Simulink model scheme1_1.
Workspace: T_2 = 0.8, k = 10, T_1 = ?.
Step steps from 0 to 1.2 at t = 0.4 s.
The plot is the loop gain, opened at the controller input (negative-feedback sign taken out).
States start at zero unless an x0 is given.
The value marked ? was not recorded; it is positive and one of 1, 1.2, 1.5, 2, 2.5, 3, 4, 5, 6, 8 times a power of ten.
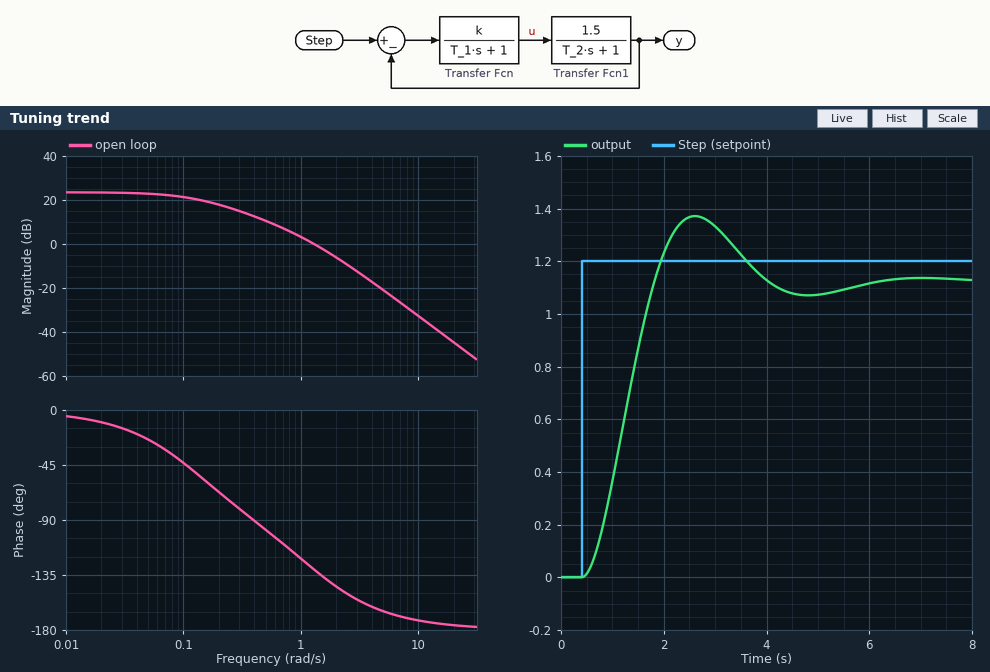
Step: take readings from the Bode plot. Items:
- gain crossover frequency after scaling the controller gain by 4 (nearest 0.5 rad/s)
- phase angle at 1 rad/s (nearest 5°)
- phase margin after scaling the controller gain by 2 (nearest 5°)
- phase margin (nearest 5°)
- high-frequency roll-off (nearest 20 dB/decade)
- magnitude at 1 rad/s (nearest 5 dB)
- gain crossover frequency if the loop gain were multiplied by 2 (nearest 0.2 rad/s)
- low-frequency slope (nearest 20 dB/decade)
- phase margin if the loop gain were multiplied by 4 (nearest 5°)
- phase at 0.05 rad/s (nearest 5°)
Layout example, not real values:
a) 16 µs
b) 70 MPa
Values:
a) 3.0 rad/s
b) -120°
c) 35°
d) 50°
e) -40 dB/decade
f) 5 dB
g) 2.0 rad/s
h) 0 dB/decade
i) 25°
j) -25°
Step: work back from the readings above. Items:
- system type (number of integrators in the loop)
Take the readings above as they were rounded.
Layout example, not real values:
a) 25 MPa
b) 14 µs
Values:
a) 0
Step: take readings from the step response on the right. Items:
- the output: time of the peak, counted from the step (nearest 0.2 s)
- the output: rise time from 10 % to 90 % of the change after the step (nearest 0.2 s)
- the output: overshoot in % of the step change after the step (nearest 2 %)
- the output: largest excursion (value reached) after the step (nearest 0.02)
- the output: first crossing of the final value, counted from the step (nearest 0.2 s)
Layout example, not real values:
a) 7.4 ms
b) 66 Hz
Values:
a) 2.2 s
b) 1.0 s
c) 22 %
d) 1.38
e) 1.4 s
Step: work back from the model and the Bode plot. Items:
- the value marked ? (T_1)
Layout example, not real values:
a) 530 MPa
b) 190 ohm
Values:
a) 8
